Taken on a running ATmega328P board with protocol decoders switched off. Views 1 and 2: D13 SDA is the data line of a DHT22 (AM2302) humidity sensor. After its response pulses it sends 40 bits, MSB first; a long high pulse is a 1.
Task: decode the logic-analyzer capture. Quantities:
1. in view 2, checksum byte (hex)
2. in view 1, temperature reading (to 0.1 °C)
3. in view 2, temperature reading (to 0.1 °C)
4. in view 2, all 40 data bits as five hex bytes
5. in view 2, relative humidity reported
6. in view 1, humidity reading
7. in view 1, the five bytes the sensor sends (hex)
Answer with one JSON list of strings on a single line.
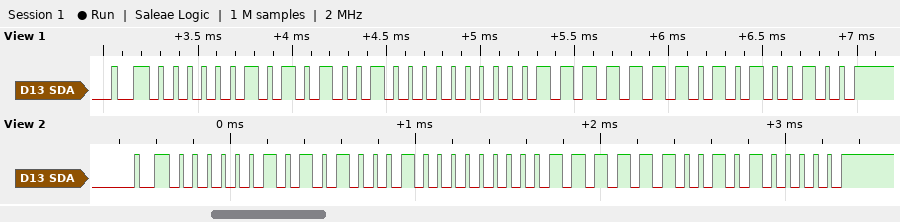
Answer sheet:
["0xA0", "25.4 °C", "25.2 °C", "02 A2 00 FC A0", "67.4 %", "67.6 %", "02 A4 00 FE A4"]
